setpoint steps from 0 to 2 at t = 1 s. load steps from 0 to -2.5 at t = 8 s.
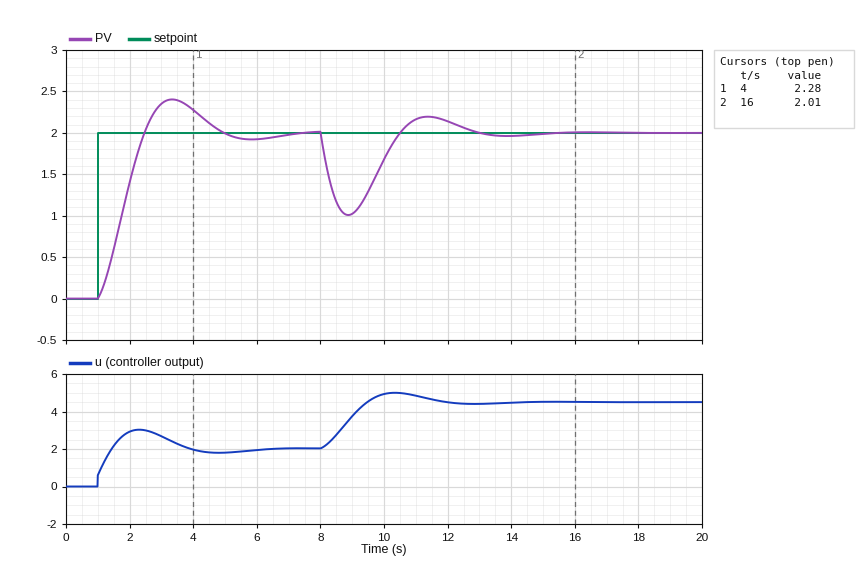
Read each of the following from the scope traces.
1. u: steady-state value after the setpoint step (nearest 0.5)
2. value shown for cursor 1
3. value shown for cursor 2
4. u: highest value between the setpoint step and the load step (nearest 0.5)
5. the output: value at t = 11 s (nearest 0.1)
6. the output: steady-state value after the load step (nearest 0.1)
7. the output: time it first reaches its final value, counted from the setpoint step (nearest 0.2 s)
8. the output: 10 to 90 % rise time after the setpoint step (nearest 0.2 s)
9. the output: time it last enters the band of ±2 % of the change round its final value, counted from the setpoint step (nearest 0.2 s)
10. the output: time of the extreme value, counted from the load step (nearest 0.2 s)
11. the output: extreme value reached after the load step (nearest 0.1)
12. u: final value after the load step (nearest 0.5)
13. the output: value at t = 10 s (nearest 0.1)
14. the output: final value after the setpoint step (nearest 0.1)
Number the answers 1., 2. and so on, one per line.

1. 2.0
2. 2.28
3. 2.01
4. 3.0
5. 2.2
6. 2.0
7. 1.4 s
8. 1.0 s
9. 5.8 s
10. 0.8 s
11. 1.0
12. 4.5
13. 1.7
14. 2.0
